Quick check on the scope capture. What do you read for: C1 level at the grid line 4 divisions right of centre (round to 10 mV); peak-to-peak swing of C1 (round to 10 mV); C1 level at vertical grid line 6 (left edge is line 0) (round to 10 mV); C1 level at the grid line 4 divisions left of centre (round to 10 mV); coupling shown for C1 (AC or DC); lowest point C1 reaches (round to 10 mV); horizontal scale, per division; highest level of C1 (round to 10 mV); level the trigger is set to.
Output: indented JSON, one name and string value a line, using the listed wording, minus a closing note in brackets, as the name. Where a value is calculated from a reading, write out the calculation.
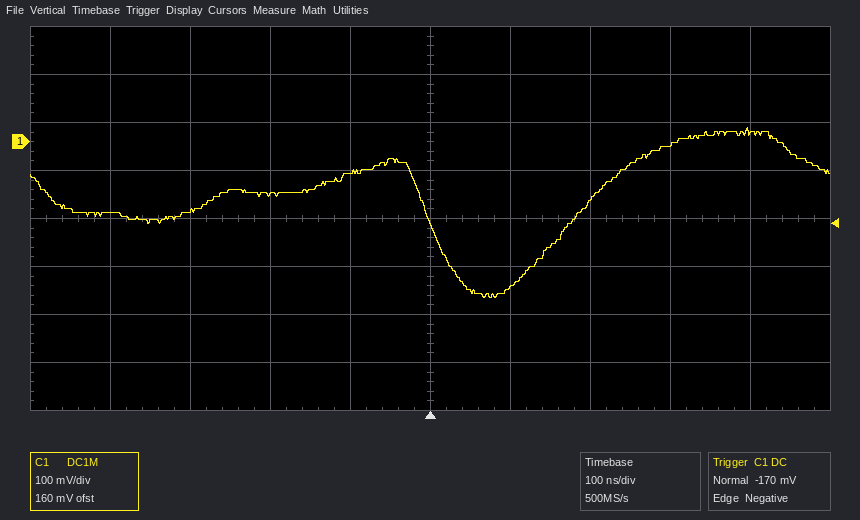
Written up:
{
  "C1 level at the grid line 4 divisions right of centre": "20 mV",
  "peak-to-peak swing of C1": "30 mV − (-320 mV) = 350 mV",
  "C1 level at vertical grid line 6 (left edge is line 0)": "-300 mV",
  "C1 level at the grid line 4 divisions left of centre": "-150 mV",
  "coupling shown for C1": "DC",
  "lowest point C1 reaches": "-320 mV",
  "horizontal scale, per division": "100 ns",
  "highest level of C1": "30 mV",
  "level the trigger is set to": "-170 mV"
}
